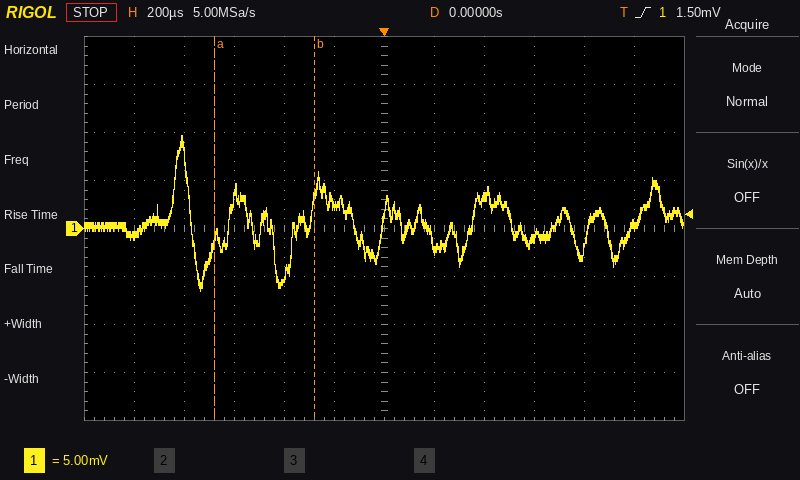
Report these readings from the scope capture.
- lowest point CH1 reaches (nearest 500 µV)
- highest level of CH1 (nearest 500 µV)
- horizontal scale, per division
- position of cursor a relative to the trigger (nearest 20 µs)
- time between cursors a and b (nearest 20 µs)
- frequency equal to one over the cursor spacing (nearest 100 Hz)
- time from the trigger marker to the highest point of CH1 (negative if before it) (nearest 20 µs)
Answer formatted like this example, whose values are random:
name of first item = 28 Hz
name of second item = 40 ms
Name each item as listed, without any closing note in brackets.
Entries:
lowest point CH1 reaches = -6.5 mV
highest level of CH1 = 9.5 mV
horizontal scale, per division = 200 µs
position of cursor a relative to the trigger = -680 µs
time between cursors a and b = 400 µs
frequency equal to one over the cursor spacing = 2.5 kHz
time from the trigger marker to the highest point of CH1 (negative if before it) = -800 µs
